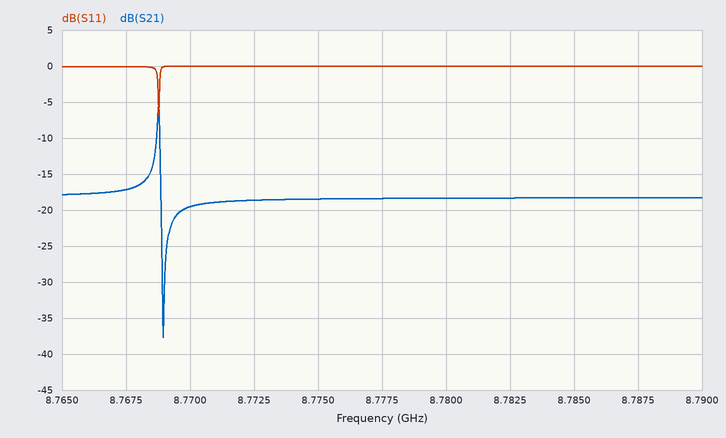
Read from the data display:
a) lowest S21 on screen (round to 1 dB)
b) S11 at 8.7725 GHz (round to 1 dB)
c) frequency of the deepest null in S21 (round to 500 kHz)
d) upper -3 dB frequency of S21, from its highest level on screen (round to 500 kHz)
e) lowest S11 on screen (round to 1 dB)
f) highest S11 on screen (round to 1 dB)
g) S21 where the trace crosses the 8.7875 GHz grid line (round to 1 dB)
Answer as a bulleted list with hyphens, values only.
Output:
- -38 dB
- 0 dB
- 8.7690 GHz
- 8.7690 GHz
- -7 dB
- 0 dB
- -18 dB
